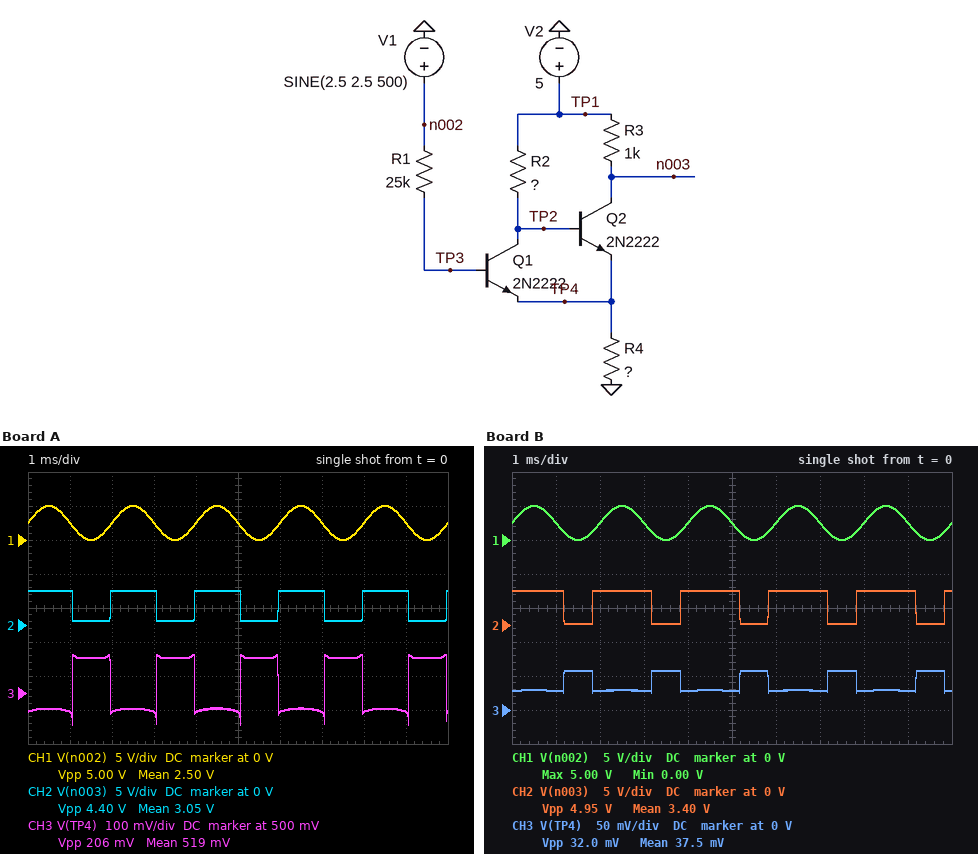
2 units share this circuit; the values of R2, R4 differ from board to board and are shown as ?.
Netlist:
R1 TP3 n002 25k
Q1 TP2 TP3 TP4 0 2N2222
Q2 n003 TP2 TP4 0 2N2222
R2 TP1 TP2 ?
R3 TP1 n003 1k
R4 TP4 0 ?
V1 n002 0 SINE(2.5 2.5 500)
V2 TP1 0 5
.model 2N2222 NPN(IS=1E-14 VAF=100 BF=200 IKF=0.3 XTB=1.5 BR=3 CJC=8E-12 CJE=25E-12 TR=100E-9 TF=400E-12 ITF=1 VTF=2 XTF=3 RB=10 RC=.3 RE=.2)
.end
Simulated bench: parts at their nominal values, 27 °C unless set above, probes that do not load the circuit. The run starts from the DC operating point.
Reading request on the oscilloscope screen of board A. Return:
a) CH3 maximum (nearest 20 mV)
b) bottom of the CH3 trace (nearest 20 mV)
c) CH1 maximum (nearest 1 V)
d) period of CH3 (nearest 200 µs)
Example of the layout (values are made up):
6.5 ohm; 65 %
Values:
620 mV; 400 mV; 5 V; 2.0 ms
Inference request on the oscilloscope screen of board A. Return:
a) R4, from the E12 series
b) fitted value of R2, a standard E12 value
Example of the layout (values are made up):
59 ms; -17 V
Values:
56 Ω; 560 Ω
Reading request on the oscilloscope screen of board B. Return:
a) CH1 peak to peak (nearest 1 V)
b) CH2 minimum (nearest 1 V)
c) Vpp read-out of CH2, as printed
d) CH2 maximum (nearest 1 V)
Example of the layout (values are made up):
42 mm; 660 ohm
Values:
5 V; 0 V; 4.95 V; 5 V
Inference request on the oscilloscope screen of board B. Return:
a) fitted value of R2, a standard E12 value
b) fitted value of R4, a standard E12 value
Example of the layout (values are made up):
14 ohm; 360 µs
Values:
1.2 kΩ; 6.8 Ω
